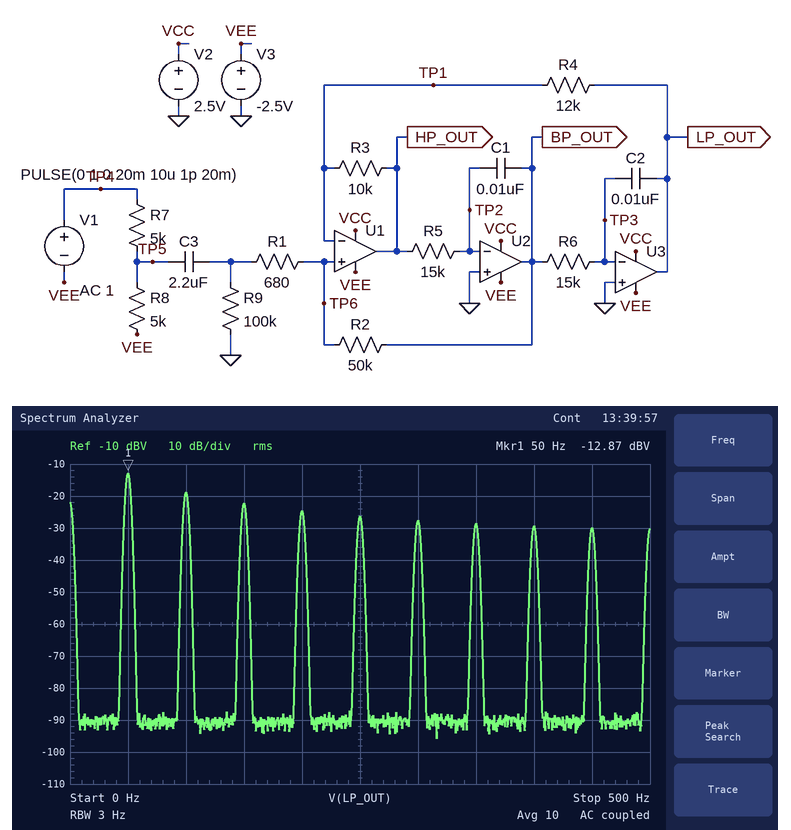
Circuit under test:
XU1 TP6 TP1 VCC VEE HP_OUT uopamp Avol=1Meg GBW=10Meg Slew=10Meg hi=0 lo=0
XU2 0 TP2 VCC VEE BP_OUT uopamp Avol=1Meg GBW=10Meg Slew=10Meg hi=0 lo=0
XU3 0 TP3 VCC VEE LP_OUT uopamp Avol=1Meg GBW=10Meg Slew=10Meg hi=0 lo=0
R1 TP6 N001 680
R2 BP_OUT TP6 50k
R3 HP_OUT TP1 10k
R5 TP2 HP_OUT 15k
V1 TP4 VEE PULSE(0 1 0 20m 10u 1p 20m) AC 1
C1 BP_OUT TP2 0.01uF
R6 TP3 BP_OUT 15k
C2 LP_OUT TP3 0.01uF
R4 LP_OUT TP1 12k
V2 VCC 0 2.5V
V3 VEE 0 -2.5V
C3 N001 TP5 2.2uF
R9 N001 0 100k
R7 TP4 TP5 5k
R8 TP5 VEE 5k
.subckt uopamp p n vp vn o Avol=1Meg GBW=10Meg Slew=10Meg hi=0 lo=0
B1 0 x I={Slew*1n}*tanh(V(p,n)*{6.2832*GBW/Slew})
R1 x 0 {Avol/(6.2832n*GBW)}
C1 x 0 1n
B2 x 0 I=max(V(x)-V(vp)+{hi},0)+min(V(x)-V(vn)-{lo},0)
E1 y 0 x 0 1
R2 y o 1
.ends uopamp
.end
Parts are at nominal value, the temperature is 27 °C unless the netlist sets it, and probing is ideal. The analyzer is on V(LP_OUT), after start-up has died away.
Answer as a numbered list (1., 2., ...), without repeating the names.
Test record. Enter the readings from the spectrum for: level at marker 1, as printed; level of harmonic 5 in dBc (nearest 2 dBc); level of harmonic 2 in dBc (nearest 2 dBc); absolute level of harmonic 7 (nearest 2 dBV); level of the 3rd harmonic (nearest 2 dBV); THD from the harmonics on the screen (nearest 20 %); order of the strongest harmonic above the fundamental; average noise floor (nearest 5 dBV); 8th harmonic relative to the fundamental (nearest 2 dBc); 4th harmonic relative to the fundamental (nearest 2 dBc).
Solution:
1. -12.87 dBV
2. -14 dBc
3. -6 dBc
4. -28 dBV
5. -22 dBV
6. 80 %
7. 2
8. -90 dBV
9. -16 dBc
10. -12 dBc
